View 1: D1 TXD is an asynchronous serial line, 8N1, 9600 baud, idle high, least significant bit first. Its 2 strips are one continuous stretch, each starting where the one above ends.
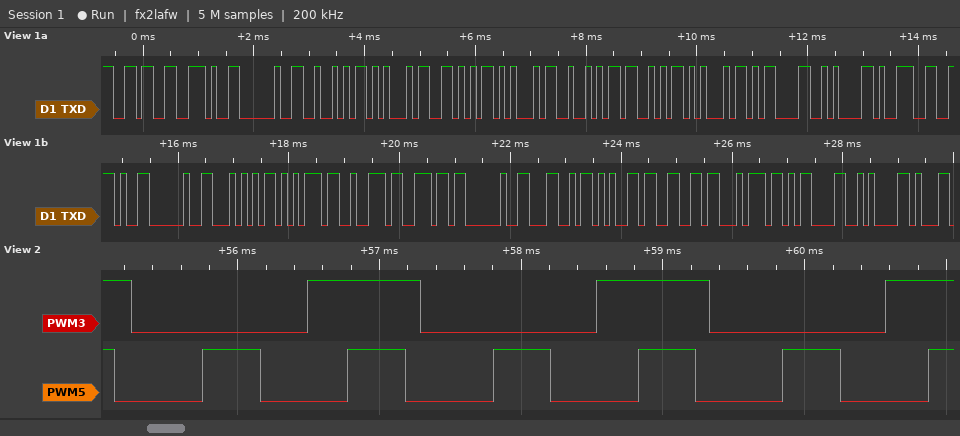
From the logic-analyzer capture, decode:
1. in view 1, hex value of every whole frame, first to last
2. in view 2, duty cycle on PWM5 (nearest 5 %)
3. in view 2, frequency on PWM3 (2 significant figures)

0x36 0x2E 0x20 0x52 0x45 0x56 0x45 0x52 0x53 0x45 0x0D 0x0A 0x39 0x2E 0x20 0x54 0x75 0x72 0x6E 0x20 0x4C 0x65 0x66 0x74 0x0D 0x0A
40 %
490 Hz
